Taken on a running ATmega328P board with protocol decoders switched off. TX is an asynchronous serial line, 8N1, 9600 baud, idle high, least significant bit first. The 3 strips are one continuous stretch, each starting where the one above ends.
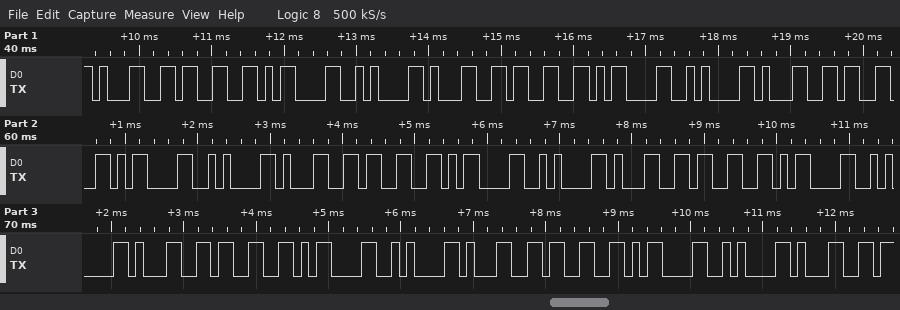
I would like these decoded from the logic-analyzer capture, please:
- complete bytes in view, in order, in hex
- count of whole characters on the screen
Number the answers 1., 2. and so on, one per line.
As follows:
1. 0x31 0x33 0x0D 0x0A 0x31 0x33 0x0D 0x0A 0x31 0x33 0x0D 0x0A 0x31 0x33 0x0D 0x0A 0x31 0x33 0x0D 0x0A 0x31 0x33 0x0D 0x0A 0x31 0x33 0x0D 0x0A 0x31
2. 29
